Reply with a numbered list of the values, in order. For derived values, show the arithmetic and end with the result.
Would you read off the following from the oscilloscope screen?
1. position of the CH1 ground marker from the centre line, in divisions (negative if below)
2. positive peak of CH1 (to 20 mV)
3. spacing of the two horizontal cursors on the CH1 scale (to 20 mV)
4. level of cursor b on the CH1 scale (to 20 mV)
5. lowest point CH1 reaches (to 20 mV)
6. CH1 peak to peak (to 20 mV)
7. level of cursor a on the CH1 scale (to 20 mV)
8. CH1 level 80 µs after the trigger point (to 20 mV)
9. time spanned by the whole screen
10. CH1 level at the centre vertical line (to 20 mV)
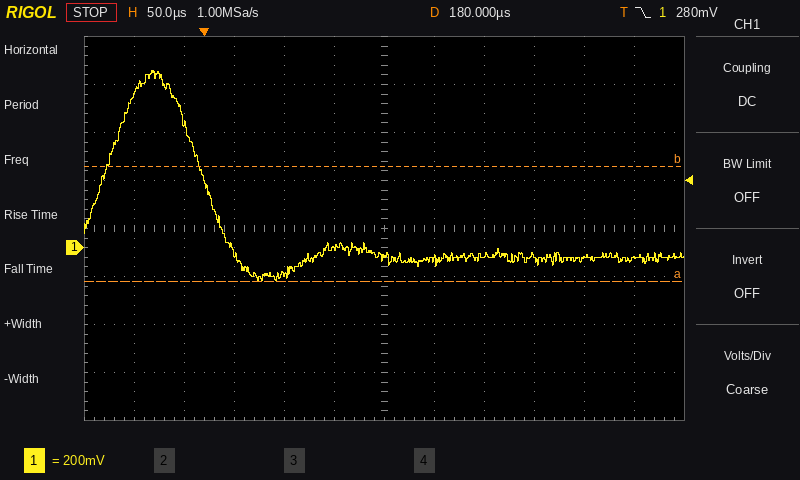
1. -0.4 div
2. 740 mV
3. 480 mV
4. 340 mV
5. -140 mV
6. 740 mV − (-140 mV) = 880 mV
7. -140 mV
8. -120 mV
9. 600 µs
10. -40 mV
